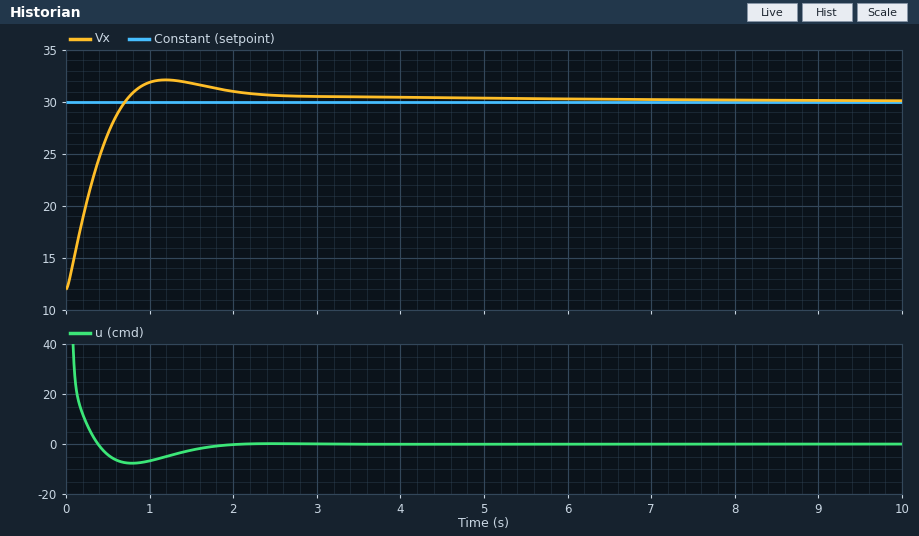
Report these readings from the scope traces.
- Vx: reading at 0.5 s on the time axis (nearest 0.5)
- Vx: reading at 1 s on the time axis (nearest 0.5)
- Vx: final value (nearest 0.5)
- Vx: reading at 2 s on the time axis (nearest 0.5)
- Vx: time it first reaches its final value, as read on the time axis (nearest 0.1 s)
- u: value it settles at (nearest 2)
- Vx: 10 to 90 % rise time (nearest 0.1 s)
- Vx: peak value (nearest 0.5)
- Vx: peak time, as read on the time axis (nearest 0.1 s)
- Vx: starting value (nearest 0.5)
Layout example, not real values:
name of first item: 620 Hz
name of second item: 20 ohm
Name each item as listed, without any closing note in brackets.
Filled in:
Vx: reading at 0.5 s on the time axis: 27.0
Vx: reading at 1 s on the time axis: 32.0
Vx: final value: 30.0
Vx: reading at 2 s on the time axis: 31.0
Vx: time it first reaches its final value, as read on the time axis: 0.7 s
u: value it settles at: 0
Vx: 10 to 90 % rise time: 0.5 s
Vx: peak value: 32.0
Vx: peak time, as read on the time axis: 1.2 s
Vx: starting value: 12.0
